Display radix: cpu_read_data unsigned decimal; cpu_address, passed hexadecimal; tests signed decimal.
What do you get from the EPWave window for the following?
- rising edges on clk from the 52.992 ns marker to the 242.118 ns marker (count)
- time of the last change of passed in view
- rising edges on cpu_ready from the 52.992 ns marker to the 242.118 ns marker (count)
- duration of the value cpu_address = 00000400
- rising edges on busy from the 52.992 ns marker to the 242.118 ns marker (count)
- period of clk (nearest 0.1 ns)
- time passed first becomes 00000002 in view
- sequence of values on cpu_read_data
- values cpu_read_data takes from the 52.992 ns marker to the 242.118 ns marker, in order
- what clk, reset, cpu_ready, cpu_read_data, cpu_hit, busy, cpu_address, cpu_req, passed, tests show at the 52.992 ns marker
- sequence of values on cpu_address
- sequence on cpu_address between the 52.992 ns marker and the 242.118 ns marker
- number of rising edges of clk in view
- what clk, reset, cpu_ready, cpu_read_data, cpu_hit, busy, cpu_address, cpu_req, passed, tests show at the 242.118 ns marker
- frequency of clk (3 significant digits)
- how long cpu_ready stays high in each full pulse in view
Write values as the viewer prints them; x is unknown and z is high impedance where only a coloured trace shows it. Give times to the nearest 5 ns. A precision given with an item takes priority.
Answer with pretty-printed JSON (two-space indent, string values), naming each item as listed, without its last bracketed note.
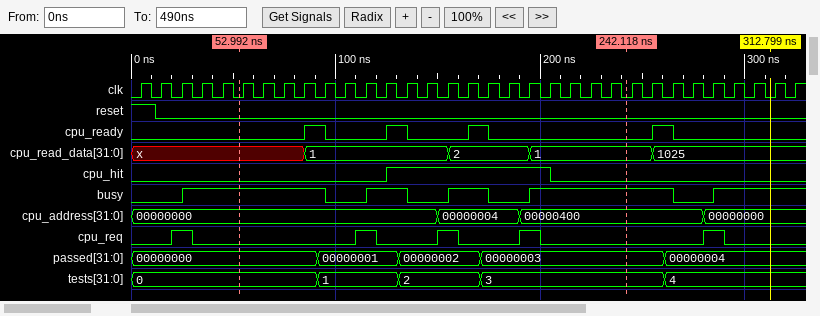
{
  "rising edges on clk from the 52.992 ns marker to the 242.118 ns marker": "19",
  "time of the last change of passed in view": "260 ns",
  "rising edges on cpu_ready from the 52.992 ns marker to the 242.118 ns marker": "3",
  "duration of the value cpu_address = 00000400": "90 ns",
  "rising edges on busy from the 52.992 ns marker to the 242.118 ns marker": "3",
  "period of clk": "10 ns",
  "time passed first becomes 00000002 in view": "130 ns",
  "sequence of values on cpu_read_data": "x, 1, 2, 1, 1025",
  "values cpu_read_data takes from the 52.992 ns marker to the 242.118 ns marker, in order": "x, 1, 2, 1",
  "what clk, reset, cpu_ready, cpu_read_data, cpu_hit, busy, cpu_address, cpu_req, passed, tests show at the 52.992 ns marker": "clk=0, reset=0, cpu_ready=0, cpu_read_data=x, cpu_hit=0, busy=1, cpu_address=00000000, cpu_req=0, passed=00000000, tests=0",
  "sequence of values on cpu_address": "00000000, 00000004, 00000400, 00000000",
  "sequence on cpu_address between the 52.992 ns marker and the 242.118 ns marker": "00000000, 00000004, 00000400",
  "number of rising edges of clk in view": "33",
  "what clk, reset, cpu_ready, cpu_read_data, cpu_hit, busy, cpu_address, cpu_req, passed, tests show at the 242.118 ns marker": "clk=0, reset=0, cpu_ready=0, cpu_read_data=1, cpu_hit=0, busy=1, cpu_address=00000400, cpu_req=0, passed=00000003, tests=3",
  "frequency of clk": "100 MHz",
  "how long cpu_ready stays high in each full pulse in view": "10 ns, 10 ns, 10 ns, 10 ns"
}
